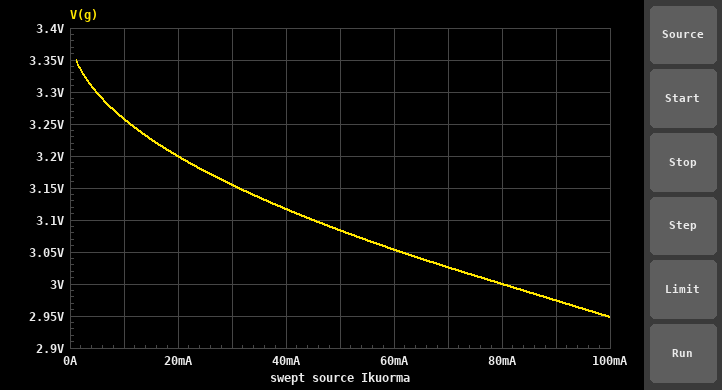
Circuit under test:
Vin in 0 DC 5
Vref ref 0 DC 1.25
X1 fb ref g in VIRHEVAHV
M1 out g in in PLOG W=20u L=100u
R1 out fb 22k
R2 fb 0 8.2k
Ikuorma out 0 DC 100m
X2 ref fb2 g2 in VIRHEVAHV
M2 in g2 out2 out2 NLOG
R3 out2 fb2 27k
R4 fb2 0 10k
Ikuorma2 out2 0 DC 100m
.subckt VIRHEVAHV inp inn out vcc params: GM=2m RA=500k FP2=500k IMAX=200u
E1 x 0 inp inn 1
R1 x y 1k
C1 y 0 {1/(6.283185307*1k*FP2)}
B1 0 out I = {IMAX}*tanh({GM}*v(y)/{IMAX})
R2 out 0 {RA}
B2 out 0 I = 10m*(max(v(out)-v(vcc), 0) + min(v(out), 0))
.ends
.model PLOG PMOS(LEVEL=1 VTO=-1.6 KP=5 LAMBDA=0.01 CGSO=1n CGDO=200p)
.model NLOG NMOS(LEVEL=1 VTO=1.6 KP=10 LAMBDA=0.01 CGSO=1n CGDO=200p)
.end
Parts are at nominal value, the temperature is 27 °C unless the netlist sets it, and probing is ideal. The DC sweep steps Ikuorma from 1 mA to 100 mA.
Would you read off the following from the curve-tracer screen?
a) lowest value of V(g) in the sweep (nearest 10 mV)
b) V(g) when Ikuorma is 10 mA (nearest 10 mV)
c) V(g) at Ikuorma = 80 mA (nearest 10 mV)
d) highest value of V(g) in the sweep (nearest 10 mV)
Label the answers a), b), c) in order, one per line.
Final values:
a) 2.95 V
b) 3.26 V
c) 3.00 V
d) 3.35 V
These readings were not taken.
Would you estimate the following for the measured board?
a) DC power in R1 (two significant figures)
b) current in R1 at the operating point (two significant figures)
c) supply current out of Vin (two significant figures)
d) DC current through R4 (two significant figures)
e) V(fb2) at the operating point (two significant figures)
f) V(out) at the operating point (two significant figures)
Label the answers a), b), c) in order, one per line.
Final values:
a) 510 µW
b) 150 µA
c) 200 mA
d) 89 µA
e) 890 mV
f) 4.6 V
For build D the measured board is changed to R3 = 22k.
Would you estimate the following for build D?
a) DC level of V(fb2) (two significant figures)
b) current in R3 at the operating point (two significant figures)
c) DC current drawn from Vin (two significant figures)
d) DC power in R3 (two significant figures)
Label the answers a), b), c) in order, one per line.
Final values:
a) 1.0 V
b) 100 µA
c) 200 mA
d) 230 µW
